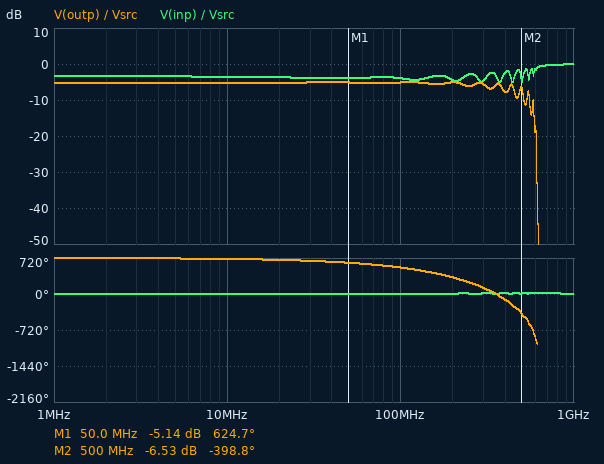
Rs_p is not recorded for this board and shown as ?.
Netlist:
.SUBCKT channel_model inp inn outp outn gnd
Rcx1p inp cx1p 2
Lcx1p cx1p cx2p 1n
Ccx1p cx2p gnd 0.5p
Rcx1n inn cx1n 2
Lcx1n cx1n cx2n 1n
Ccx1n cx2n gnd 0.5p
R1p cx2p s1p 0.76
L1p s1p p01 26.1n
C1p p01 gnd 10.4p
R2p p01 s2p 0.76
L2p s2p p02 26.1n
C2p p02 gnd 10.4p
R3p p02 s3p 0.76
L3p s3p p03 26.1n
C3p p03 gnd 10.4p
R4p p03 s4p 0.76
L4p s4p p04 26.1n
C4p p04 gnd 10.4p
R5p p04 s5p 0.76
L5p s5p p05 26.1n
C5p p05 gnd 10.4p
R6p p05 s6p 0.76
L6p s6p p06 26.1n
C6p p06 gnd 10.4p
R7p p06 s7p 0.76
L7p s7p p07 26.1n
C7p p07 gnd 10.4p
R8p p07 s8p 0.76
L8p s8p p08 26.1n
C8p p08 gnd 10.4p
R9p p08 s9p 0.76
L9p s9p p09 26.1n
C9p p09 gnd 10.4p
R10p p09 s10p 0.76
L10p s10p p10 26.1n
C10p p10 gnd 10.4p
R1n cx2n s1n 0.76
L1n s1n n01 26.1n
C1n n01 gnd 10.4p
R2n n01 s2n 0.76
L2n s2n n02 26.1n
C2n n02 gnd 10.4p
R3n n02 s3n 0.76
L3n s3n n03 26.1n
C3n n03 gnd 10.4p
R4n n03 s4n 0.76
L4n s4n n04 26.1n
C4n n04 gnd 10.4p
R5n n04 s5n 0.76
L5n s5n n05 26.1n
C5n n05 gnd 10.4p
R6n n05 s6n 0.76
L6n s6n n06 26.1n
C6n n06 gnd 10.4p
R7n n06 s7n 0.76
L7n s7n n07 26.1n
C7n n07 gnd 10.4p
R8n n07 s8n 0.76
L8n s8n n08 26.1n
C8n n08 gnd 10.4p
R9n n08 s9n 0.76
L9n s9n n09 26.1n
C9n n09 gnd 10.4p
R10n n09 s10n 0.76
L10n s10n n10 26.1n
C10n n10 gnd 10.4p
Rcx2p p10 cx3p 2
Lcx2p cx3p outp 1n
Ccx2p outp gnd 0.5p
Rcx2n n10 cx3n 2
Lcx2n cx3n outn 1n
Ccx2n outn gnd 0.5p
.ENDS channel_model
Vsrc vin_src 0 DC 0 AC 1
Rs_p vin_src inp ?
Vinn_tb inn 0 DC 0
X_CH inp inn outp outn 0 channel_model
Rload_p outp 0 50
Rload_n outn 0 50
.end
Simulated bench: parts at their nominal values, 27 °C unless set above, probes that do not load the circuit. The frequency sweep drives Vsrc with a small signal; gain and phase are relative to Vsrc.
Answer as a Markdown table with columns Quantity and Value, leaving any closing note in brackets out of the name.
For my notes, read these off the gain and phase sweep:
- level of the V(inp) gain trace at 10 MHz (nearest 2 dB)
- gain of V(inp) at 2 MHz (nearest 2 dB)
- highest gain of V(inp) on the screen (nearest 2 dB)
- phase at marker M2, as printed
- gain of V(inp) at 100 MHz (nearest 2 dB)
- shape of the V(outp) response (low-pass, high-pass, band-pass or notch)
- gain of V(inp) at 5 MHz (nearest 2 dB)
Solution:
| Quantity | Value |
|---|---|
| level of the V(inp) gain trace at 10 MHz | -4 dB |
| gain of V(inp) at 2 MHz | -4 dB |
| highest gain of V(inp) on the screen | 0 dB |
| phase at marker M2, as printed | -398.8 deg |
| gain of V(inp) at 100 MHz | -4 dB |
| shape of the V(outp) response | low-pass |
| gain of V(inp) at 5 MHz | -4 dB |
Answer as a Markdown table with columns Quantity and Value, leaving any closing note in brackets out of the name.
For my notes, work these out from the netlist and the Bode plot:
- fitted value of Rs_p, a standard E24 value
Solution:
| Quantity | Value |
|---|---|
| fitted value of Rs_p, a standard E24 value | 30 Ω |
